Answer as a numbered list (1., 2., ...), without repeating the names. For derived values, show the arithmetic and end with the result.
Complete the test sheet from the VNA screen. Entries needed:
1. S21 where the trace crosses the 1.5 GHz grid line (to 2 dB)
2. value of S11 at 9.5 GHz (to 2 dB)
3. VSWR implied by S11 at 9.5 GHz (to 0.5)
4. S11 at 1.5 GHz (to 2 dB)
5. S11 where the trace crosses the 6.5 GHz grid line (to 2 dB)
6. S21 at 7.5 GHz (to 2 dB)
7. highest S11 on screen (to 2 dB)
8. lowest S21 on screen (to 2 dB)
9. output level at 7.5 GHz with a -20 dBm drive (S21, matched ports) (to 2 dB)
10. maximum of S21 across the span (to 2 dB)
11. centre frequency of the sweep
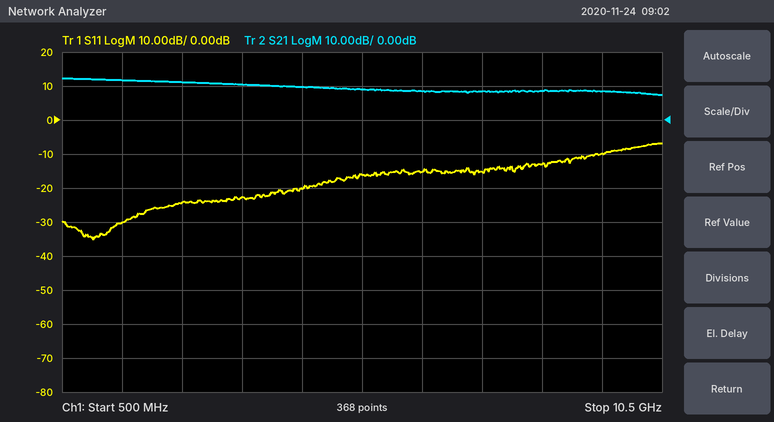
1. 12 dB
2. -10 dB
3. |Γ| = 10^(-10/20) = 0.3162; VSWR = (1 + 0.3162)/(1 − 0.3162) ≈ 1.92, so 2.0 to the nearest 0.5
4. -30 dB
5. -16 dB
6. 8 dB
7. -6 dB
8. 8 dB
9. -20 dBm + (8 dB) = -12 dBm
10. 12 dB
11. 5.5 GHz
